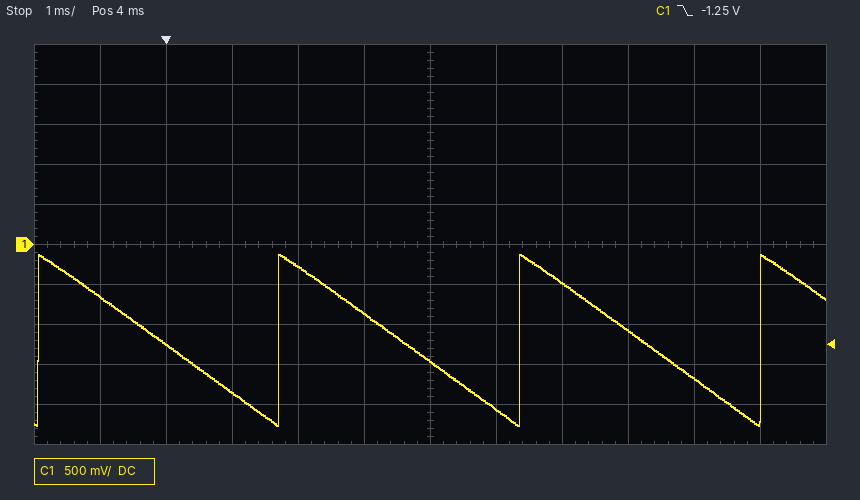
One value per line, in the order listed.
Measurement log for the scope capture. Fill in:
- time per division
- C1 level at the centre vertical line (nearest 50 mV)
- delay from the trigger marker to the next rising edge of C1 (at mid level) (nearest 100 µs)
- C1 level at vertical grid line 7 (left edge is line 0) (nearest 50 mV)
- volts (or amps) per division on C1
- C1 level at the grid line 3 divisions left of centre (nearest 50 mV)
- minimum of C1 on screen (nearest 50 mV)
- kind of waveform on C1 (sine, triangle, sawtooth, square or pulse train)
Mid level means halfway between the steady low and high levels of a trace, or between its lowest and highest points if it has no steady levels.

1 ms
-1.45 V
1.7 ms
-2.05 V
500 mV
-1.85 V
-2.25 V
sawtooth
